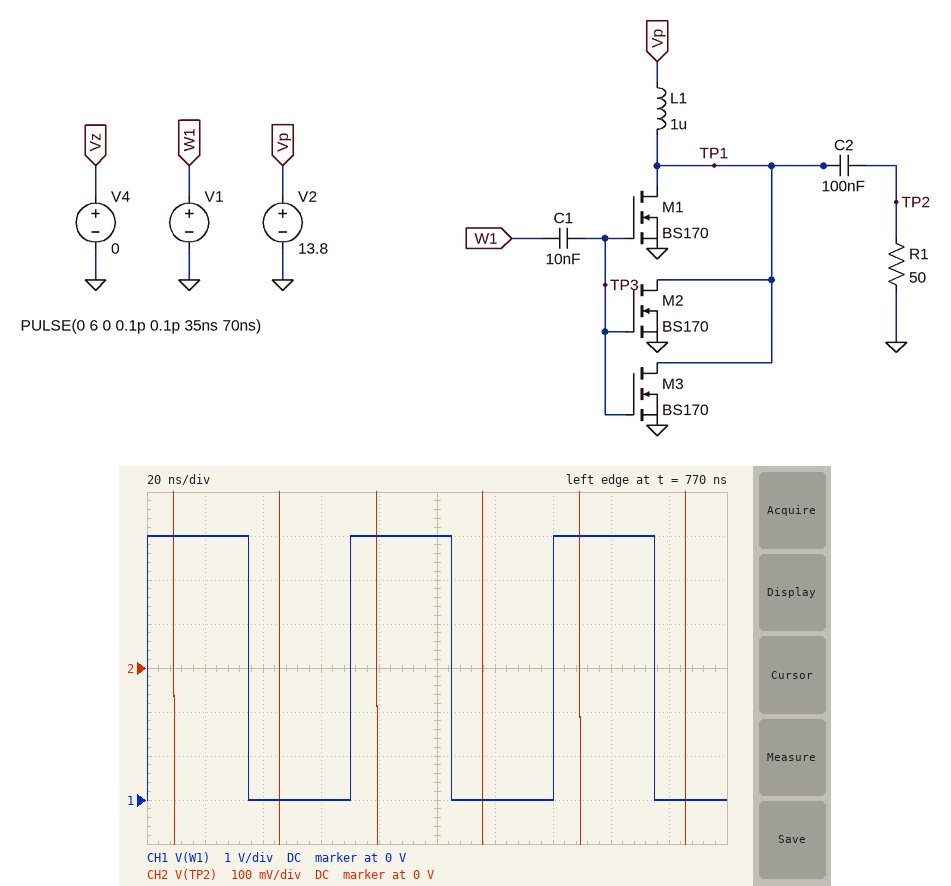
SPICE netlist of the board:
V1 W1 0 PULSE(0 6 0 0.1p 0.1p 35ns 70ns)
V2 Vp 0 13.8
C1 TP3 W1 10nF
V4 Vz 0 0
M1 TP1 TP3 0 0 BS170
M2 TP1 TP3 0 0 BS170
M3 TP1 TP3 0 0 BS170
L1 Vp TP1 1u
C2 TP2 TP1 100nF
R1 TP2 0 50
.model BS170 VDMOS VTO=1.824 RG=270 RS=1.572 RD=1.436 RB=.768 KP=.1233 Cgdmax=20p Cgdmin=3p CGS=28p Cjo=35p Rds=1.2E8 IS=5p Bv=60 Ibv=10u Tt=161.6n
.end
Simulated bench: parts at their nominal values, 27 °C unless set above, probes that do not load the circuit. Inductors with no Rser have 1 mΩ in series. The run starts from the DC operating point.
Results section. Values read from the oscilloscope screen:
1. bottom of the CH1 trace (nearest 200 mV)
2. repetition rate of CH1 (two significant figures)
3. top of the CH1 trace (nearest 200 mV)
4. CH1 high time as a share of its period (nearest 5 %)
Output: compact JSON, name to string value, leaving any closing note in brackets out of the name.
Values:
{"bottom of the CH1 trace": "0 V", "repetition rate of CH1": "14 MHz", "top of the CH1 trace": "6.0 V", "CH1 high time as a share of its period": "50 %"}
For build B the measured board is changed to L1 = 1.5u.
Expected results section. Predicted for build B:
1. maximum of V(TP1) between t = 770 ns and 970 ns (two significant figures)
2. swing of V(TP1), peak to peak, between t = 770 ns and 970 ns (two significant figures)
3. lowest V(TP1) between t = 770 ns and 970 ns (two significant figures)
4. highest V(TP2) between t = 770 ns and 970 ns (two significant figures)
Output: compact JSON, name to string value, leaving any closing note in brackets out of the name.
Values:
{"maximum of V(TP1) between t = 770 ns and 970 ns": "31 V", "swing of V(TP1), peak to peak, between t = 770 ns and 970 ns": "30 V", "lowest V(TP1) between t = 770 ns and 970 ns": "1.2 V", "highest V(TP2) between t = 770 ns and 970 ns": "19 V"}
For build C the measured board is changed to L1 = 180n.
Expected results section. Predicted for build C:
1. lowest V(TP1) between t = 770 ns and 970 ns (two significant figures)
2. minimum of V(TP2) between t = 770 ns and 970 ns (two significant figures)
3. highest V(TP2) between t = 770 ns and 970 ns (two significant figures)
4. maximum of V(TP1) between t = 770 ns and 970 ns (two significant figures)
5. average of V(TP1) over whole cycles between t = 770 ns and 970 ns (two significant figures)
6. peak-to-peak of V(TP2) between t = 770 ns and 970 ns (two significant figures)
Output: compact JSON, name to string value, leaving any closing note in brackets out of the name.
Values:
{"lowest V(TP1) between t = 770 ns and 970 ns": "3.1 V", "minimum of V(TP2) between t = 770 ns and 970 ns": "-9.1 V", "highest V(TP2) between t = 770 ns and 970 ns": "30 V", "maximum of V(TP1) between t = 770 ns and 970 ns": "42 V", "average of V(TP1) over whole cycles between t = 770 ns and 970 ns": "14 V", "peak-to-peak of V(TP2) between t = 770 ns and 970 ns": "39 V"}
